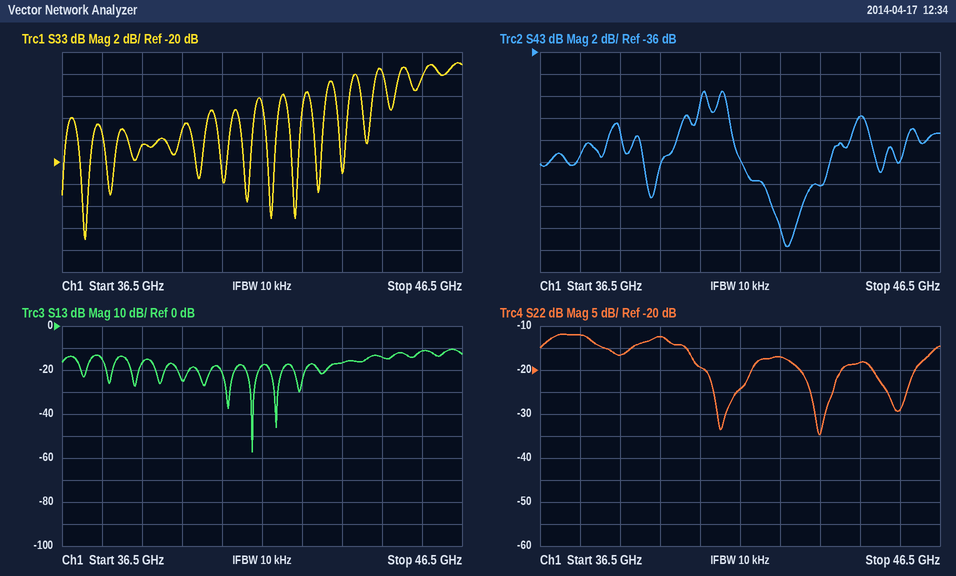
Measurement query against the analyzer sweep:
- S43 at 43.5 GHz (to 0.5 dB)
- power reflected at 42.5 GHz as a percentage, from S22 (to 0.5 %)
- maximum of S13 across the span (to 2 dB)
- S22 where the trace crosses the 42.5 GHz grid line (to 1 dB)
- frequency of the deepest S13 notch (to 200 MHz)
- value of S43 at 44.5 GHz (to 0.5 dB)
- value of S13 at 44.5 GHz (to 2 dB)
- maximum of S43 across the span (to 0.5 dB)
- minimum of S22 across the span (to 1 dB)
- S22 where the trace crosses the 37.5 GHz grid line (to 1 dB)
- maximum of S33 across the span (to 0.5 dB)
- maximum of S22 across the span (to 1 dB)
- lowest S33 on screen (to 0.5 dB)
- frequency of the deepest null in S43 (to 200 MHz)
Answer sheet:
-48.0 dB
2.0 %
-10 dB
-17 dB
41.2 GHz
-42.0 dB
-14 dB
-39.5 dB
-35 dB
-12 dB
-11.0 dB
-12 dB
-27.0 dB
42.6 GHz
